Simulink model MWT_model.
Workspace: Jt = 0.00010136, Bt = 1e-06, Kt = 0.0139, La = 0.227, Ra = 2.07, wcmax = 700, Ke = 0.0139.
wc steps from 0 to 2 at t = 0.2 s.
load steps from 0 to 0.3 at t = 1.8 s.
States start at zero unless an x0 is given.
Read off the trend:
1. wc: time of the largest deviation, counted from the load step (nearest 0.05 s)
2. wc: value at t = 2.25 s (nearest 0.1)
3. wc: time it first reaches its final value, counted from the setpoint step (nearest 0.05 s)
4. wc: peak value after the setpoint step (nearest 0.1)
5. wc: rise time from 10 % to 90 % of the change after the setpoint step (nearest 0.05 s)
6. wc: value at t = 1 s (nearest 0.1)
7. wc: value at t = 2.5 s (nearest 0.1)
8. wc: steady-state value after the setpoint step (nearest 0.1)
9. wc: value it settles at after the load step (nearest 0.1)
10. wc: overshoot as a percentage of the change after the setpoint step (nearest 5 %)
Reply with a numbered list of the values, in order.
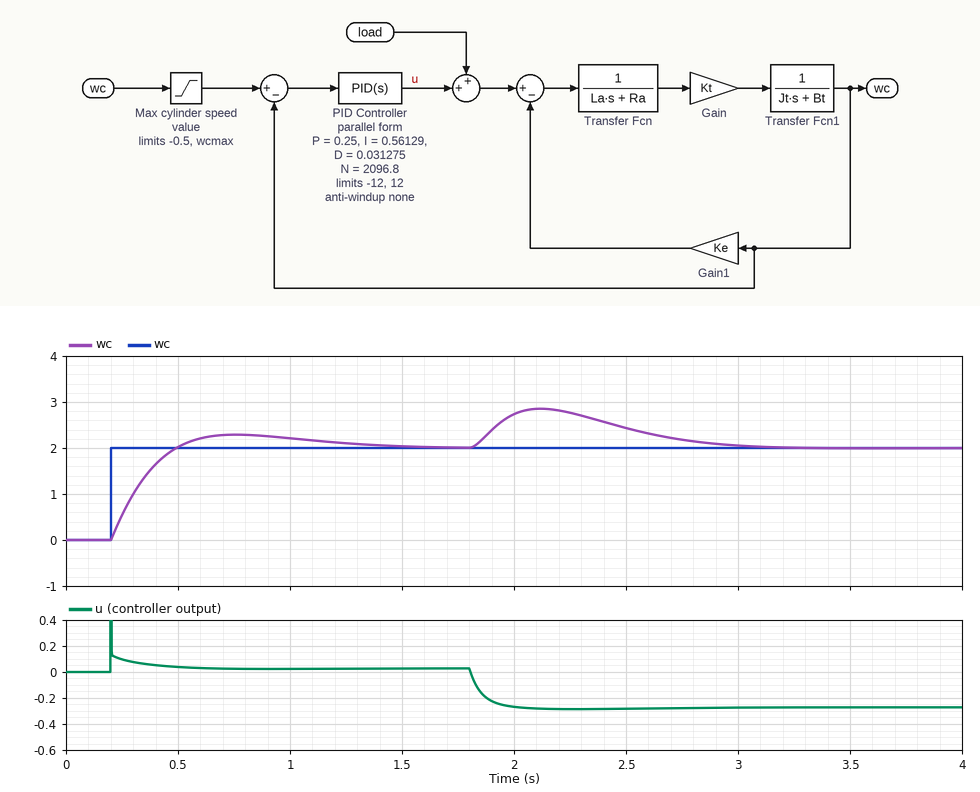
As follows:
1. 0.30 s
2. 2.8
3. 0.30 s
4. 2.3
5. 0.20 s
6. 2.2
7. 2.4
8. 2.0
9. 2.0
10. 15 %
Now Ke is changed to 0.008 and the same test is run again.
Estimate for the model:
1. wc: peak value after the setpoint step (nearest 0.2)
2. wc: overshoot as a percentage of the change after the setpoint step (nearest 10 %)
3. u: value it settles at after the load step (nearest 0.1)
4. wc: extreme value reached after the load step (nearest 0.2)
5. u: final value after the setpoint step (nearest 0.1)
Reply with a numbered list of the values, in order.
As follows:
1. 2.4
2. 20 %
3. -0.3
4. 2.8
5. 0.0
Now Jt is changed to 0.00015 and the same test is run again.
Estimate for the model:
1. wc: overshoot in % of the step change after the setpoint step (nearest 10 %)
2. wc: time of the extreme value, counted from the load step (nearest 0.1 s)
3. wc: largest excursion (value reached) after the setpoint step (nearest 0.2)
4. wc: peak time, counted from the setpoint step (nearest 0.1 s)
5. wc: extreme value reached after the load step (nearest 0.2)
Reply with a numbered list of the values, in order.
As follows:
1. 20 %
2. 0.4 s
3. 2.4
4. 0.6 s
5. 2.8
